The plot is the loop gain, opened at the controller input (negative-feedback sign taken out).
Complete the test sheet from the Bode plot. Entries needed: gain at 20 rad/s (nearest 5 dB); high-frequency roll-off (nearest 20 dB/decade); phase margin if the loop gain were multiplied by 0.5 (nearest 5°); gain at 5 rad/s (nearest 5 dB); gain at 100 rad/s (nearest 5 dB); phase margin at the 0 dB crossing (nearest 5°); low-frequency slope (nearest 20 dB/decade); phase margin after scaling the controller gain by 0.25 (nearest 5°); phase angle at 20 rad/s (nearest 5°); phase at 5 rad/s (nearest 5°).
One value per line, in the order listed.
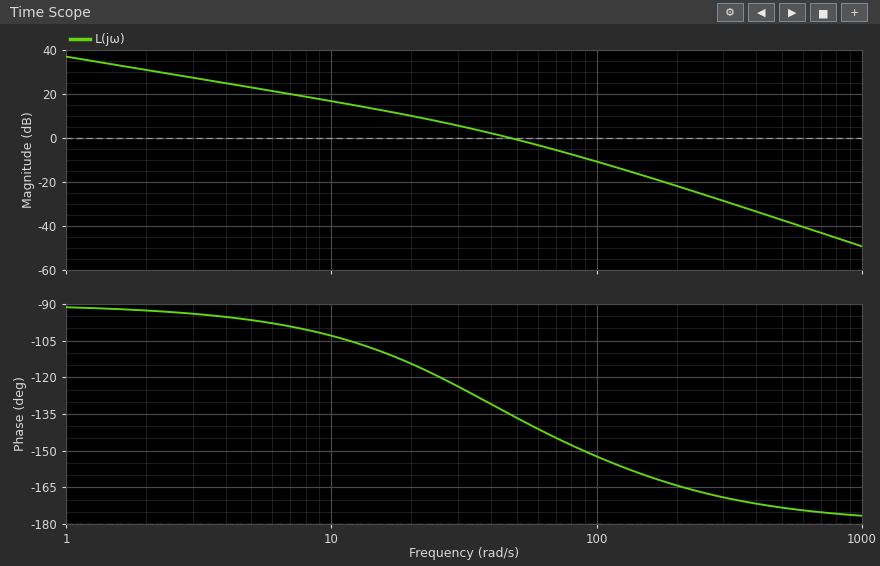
10 dB
-40 dB/decade
55°
25 dB
-10 dB
45°
-20 dB/decade
70°
-115°
-95°
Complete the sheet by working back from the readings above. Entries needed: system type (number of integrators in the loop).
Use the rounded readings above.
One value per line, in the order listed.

1
